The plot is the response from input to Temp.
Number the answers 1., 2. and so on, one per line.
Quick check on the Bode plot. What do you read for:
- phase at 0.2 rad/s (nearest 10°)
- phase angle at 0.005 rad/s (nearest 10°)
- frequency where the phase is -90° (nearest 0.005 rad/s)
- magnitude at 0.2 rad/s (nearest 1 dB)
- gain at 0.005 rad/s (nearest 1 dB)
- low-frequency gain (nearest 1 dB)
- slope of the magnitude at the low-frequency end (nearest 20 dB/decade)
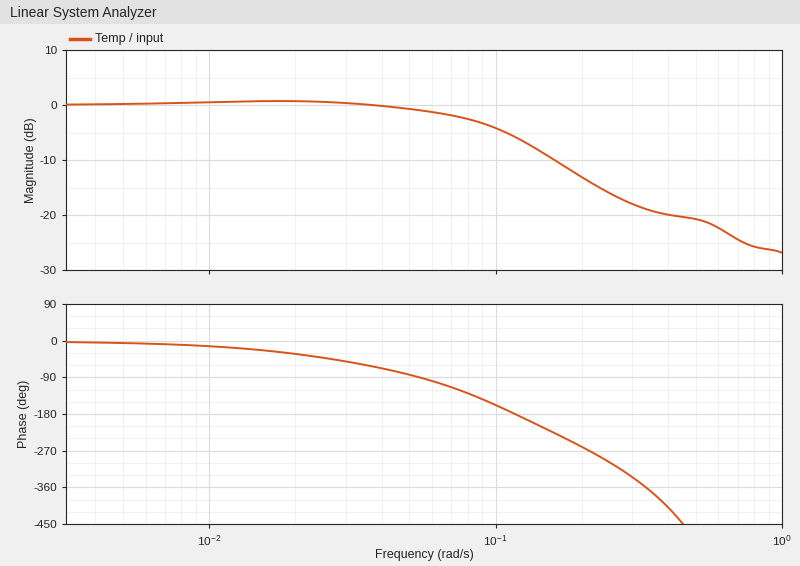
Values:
1. -260°
2. -10°
3. 0.055 rad/s
4. -13 dB
5. 0 dB
6. 0 dB
7. 0 dB/decade
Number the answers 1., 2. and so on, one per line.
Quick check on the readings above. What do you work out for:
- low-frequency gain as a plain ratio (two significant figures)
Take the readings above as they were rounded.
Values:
1. 1.0
